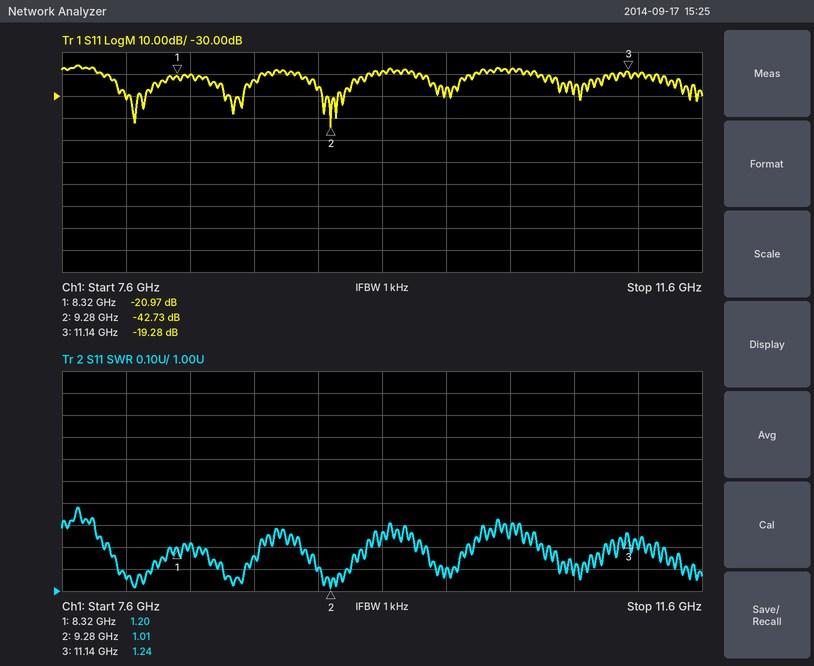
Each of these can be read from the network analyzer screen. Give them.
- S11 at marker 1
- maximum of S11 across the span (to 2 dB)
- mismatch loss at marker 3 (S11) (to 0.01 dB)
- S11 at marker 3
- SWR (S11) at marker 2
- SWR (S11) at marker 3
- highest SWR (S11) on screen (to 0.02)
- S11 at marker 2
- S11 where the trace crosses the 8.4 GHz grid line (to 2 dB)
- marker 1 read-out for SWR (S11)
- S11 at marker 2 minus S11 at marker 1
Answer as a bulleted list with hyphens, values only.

- -20.97 dB
- -16 dB
- 0.05 dB
- -19.28 dB
- 1.01
- 1.24
- 1.38
- -42.73 dB
- -20 dB
- 1.20
- -21.76 dB
